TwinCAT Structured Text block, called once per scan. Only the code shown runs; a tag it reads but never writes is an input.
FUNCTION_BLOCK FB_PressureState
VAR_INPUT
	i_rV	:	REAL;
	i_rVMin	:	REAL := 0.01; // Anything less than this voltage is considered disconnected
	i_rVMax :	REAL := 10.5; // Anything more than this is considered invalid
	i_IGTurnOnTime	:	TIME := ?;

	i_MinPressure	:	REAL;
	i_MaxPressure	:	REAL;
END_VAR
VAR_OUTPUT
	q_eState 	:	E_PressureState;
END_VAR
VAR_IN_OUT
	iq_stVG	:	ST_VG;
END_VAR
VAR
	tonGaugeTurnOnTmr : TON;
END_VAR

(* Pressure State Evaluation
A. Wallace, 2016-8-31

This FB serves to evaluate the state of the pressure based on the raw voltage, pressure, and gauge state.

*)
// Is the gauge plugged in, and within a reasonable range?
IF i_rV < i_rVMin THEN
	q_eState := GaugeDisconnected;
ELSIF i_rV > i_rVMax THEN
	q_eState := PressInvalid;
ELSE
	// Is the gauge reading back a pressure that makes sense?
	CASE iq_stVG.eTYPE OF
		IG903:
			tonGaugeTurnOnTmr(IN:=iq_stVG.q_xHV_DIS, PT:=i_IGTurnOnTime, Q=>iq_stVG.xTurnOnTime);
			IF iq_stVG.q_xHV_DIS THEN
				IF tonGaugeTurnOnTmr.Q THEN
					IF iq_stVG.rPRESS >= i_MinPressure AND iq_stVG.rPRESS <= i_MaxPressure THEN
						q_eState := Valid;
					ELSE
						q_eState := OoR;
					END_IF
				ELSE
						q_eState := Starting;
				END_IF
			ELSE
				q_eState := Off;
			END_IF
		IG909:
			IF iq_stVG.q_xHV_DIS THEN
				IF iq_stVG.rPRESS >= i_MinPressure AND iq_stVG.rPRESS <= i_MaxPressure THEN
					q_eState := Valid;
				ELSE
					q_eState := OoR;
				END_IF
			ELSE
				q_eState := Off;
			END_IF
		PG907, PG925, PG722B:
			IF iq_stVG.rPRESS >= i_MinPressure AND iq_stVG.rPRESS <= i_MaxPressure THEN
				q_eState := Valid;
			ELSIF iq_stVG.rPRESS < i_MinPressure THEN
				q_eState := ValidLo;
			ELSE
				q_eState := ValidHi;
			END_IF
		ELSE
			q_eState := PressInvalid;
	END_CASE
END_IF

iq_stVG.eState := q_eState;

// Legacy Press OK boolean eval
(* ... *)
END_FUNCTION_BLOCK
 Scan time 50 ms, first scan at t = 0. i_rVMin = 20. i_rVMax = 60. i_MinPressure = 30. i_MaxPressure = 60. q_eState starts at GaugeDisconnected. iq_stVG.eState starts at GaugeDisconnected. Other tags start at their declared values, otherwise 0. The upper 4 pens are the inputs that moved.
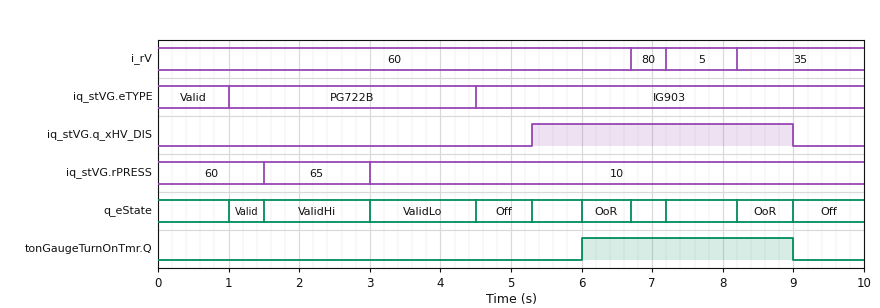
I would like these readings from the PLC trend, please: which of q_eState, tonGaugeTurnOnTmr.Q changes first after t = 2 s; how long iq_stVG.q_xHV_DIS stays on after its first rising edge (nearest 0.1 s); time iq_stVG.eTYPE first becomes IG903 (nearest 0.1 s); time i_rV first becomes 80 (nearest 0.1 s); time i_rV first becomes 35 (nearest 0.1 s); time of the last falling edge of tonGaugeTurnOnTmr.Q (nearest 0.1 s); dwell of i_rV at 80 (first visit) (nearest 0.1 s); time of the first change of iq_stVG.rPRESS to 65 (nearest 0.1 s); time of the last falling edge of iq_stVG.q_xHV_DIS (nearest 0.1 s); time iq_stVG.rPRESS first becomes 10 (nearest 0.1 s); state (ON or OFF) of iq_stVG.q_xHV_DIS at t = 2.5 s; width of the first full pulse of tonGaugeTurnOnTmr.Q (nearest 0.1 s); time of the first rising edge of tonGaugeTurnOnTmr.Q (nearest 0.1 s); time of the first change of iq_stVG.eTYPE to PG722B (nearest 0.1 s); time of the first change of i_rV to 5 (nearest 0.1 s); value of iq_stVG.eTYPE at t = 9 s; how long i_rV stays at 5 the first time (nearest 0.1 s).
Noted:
q_eState
3.7 s
4.5 s
6.7 s
8.2 s
9.0 s
0.5 s
1.5 s
9.0 s
3.0 s
OFF
3.0 s
6.0 s
1.0 s
7.2 s
IG903
1.0 s
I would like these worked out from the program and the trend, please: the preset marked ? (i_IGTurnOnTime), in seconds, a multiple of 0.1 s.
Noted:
0.7 s
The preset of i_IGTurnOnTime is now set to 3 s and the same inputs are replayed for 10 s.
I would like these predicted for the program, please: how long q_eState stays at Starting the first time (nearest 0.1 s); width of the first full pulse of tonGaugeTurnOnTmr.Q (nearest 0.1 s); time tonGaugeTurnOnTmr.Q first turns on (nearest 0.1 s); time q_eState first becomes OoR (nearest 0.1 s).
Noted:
1.4 s
0.7 s
8.3 s
8.3 s
